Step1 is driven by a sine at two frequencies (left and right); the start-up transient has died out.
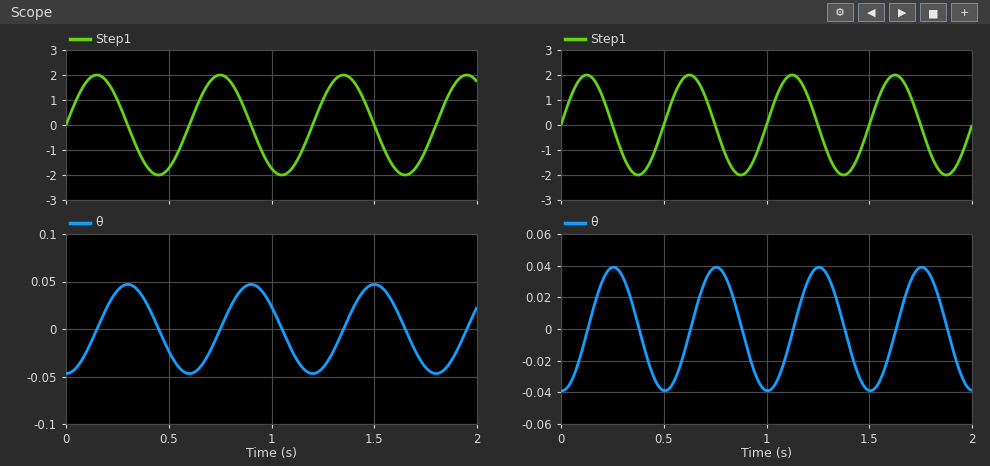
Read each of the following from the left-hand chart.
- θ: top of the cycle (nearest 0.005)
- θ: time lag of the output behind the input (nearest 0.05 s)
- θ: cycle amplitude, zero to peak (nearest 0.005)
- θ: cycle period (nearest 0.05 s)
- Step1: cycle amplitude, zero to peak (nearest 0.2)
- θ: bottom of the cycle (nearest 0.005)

0.045
0.15 s
0.045
0.60 s
2.0
-0.045
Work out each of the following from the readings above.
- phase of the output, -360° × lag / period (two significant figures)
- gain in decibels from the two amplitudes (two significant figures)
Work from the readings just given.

-90°
-33 dB
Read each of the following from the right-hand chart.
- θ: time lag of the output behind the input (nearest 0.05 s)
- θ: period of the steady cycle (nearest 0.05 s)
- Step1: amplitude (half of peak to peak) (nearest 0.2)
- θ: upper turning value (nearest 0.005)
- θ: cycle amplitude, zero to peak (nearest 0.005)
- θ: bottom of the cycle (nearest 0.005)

0.15 s
0.50 s
2.0
0.040
0.040
-0.040
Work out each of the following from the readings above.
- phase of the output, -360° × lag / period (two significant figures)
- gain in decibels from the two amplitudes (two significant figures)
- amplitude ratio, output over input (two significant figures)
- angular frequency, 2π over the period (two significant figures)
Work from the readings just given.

-110°
-34 dB
0.020
13 rad/s
